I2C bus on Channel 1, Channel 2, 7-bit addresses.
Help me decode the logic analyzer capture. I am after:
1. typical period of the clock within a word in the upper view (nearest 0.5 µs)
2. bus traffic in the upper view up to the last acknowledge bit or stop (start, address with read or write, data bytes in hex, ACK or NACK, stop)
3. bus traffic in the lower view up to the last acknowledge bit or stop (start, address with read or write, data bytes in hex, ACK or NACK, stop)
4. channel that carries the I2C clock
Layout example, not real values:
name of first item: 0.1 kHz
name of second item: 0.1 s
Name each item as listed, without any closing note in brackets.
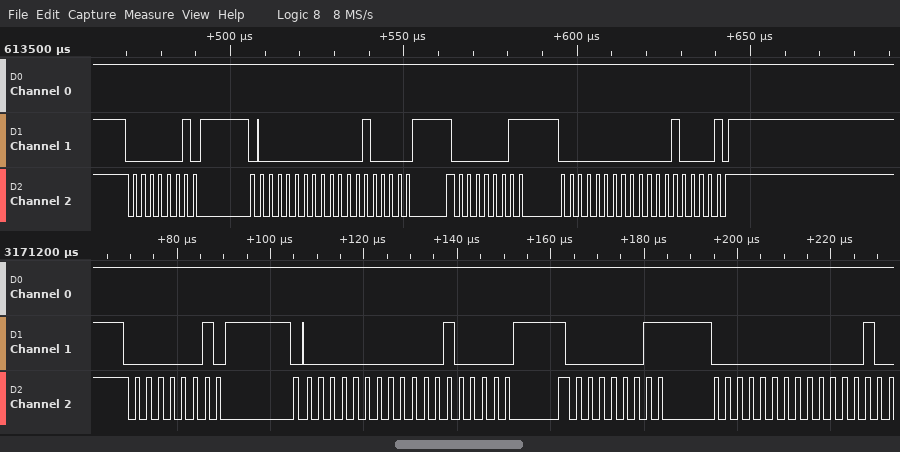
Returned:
typical period of the clock within a word in the upper view: 2.5 µs
bus traffic in the upper view up to the last acknowledge bit or stop: start, address 01 write ACK, 00 ACK, 10 ACK, repeated start, address 01 read ACK, 00 ACK, 10 NACK, stop
bus traffic in the lower view up to the last acknowledge bit or stop: start, address 01 write ACK, 00 ACK, 10 ACK, repeated start, address 01 read ACK, 00 ACK
channel that carries the I2C clock: Channel 2
